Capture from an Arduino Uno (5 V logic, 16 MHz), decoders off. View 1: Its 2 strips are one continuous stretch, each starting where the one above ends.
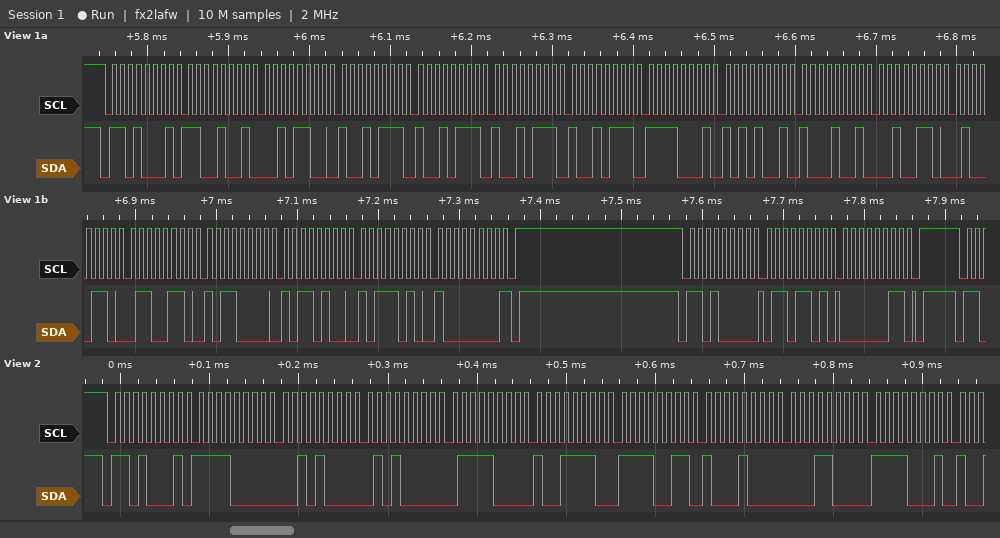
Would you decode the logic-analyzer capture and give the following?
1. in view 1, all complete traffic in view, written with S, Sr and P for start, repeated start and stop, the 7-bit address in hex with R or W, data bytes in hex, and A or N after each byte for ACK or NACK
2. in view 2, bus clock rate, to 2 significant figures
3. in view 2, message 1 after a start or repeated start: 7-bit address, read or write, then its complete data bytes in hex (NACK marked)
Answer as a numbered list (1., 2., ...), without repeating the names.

1. S 68R A C9 A 2C A 97 A 97 A 97 A 97 A F1 A A9 A 89 A 26 A 46 A 66 A B0 A B4 A BA A 80 N P S 68W A 6D A 03 A P
2. 100 kHz
3. 0x68 read: F0 28 50 78 9E F3 88 18 F1
